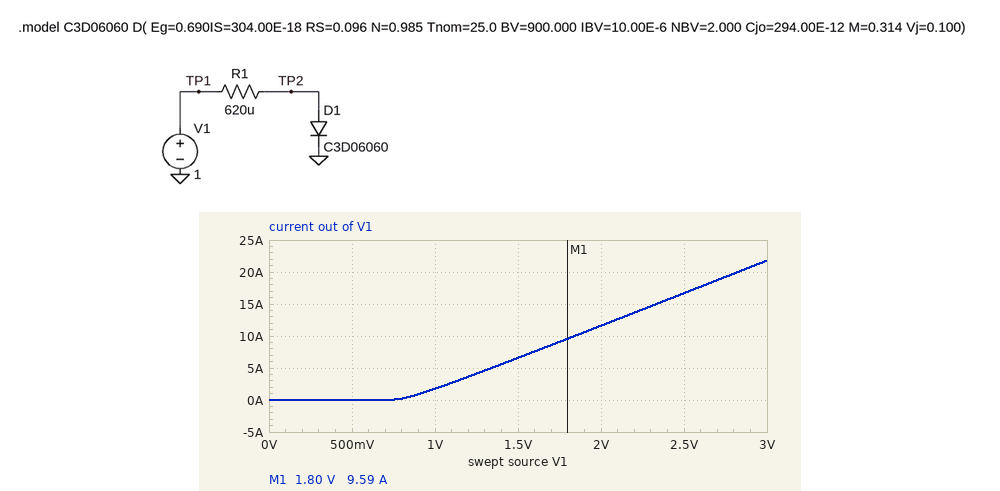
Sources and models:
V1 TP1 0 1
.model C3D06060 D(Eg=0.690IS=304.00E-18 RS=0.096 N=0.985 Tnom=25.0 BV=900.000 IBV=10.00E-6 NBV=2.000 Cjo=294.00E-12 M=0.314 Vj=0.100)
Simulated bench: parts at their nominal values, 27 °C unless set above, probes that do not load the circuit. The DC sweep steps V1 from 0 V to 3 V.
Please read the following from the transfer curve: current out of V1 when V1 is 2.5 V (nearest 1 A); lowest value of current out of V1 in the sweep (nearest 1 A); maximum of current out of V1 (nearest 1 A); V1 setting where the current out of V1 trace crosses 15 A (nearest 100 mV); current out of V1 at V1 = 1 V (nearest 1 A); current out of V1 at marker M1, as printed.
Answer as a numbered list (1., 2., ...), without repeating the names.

1. 17 A
2. 0 A
3. 22 A
4. 2.3 V
5. 2 A
6. 9.59 A
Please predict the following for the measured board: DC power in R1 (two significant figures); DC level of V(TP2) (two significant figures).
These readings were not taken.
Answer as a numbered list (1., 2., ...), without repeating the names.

1. 1.9 mW
2. 1.0 V
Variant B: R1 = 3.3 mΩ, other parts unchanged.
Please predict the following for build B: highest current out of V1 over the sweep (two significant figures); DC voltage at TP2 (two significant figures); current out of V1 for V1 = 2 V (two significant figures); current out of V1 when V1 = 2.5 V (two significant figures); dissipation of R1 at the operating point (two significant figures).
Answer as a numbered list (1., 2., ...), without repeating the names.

1. 21 A
2. 990 mV
3. 11 A
4. 16 A
5. 9.7 mW
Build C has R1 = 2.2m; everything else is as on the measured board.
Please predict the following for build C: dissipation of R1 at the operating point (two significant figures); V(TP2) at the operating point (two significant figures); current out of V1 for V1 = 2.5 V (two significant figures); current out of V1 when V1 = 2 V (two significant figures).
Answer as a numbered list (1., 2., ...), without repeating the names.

1. 6.6 mW
2. 1.0 V
3. 16 A
4. 11 A
